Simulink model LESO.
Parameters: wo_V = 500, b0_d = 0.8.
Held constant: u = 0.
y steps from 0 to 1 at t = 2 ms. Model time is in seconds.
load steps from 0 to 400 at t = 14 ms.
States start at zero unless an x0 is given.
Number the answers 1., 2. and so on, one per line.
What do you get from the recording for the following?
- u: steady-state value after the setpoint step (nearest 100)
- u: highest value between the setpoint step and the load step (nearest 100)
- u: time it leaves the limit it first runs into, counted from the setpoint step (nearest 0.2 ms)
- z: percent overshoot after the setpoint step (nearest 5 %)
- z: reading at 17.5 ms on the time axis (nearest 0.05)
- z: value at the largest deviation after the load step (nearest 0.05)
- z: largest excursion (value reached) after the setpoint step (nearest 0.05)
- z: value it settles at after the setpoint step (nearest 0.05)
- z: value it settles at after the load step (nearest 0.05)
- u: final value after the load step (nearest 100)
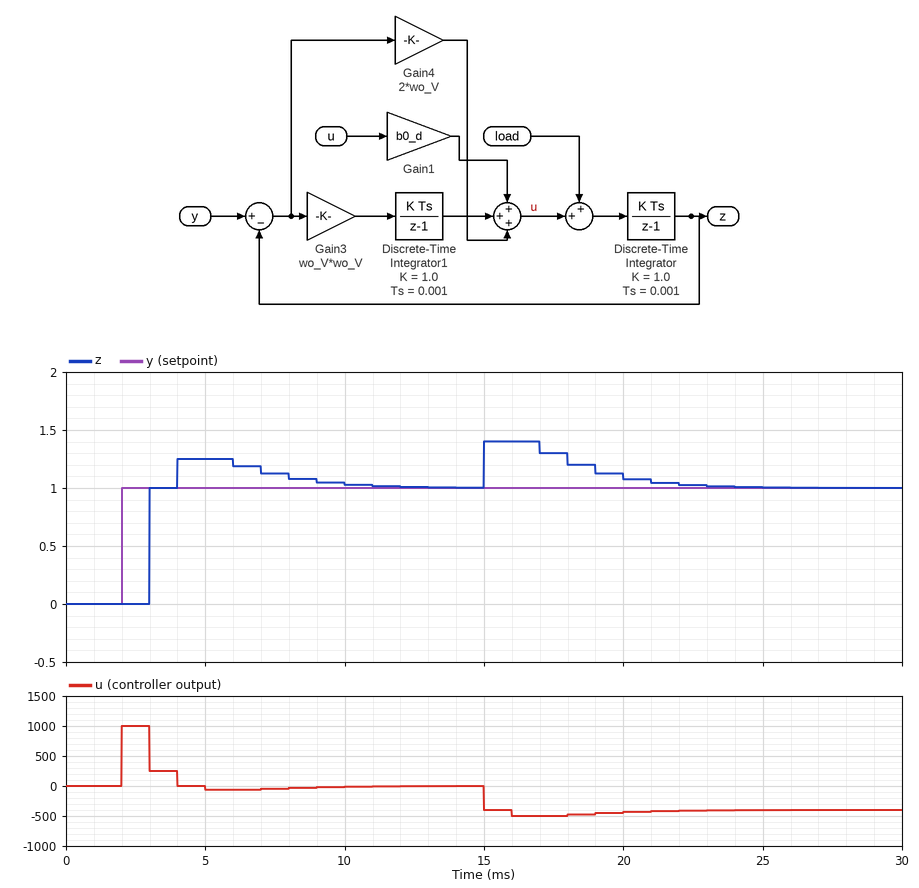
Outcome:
1. 0
2. 1000
3. 1.0 ms
4. 25 %
5. 1.30
6. 1.40
7. 1.25
8. 1.00
9. 1.00
10. -400
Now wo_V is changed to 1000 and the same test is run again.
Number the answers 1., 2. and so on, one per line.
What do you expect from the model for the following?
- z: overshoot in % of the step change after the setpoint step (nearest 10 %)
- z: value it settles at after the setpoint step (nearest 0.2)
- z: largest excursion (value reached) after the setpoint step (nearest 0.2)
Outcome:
1. 100 %
2. 1.0
3. 2.0
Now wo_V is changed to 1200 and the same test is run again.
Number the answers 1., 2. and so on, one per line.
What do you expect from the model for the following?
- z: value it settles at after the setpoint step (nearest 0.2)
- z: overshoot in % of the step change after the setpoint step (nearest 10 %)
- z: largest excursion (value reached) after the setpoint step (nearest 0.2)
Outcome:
1. 1.0
2. 140 %
3. 2.4
